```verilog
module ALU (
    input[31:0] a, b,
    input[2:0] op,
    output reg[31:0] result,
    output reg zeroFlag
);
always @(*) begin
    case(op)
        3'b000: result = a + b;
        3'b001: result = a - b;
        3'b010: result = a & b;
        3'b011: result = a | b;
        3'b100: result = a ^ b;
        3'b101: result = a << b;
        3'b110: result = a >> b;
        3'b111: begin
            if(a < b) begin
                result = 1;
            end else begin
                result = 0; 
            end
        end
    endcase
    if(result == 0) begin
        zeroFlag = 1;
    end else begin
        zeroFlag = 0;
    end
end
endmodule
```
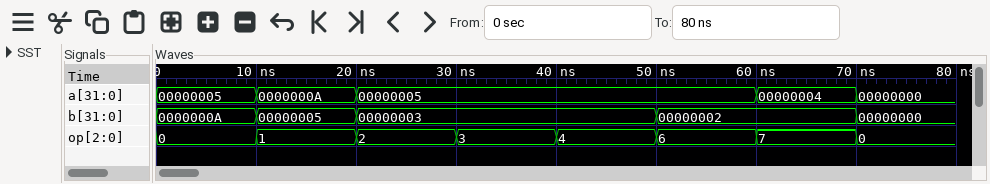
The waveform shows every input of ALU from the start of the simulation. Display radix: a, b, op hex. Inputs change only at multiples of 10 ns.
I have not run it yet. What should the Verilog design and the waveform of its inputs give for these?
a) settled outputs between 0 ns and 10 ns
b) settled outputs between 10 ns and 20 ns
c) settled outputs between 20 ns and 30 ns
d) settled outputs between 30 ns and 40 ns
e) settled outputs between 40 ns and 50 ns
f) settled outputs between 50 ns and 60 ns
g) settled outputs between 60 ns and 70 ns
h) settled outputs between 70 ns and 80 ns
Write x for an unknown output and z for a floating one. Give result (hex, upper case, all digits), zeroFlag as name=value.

result=0000000F, zeroFlag=0
result=00000005, zeroFlag=0
result=00000001, zeroFlag=0
result=00000007, zeroFlag=0
result=00000006, zeroFlag=0
result=00000001, zeroFlag=0
result=00000000, zeroFlag=1
result=00000000, zeroFlag=1
